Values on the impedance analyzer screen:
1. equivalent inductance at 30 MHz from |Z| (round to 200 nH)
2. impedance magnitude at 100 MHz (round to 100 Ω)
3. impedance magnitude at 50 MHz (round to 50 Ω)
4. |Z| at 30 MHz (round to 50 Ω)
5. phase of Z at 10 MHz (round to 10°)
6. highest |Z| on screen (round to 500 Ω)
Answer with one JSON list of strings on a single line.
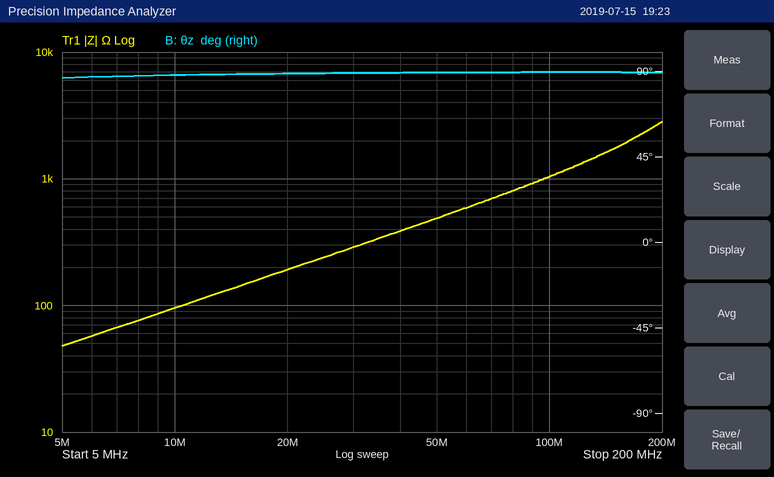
["1.6 µH", "1.0 kΩ", "500 Ω", "300 Ω", "90°", "3.0 kΩ"]
